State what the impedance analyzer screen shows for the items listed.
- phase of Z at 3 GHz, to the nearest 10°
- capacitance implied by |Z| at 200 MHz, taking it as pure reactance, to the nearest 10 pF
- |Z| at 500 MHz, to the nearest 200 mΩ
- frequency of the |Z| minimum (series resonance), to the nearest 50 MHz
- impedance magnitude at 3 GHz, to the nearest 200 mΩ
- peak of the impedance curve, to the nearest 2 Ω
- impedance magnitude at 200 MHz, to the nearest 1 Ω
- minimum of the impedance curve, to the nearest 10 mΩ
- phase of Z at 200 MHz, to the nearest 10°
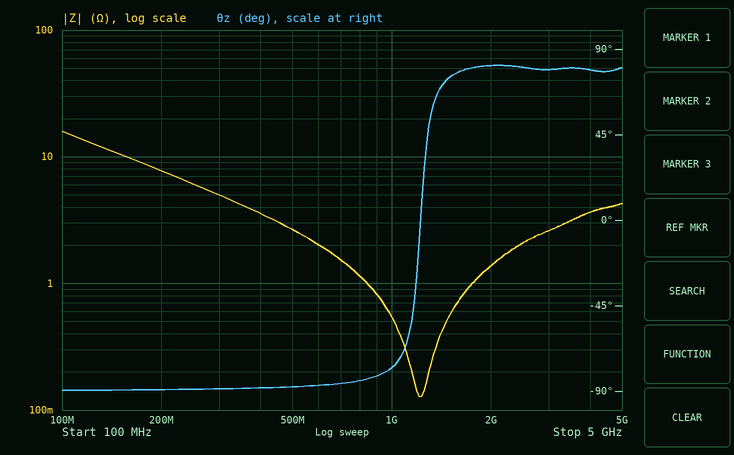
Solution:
80°
100 pF
2.6 Ω
1.20 GHz
2.6 Ω
16 Ω
8 Ω
130 mΩ
-90°
